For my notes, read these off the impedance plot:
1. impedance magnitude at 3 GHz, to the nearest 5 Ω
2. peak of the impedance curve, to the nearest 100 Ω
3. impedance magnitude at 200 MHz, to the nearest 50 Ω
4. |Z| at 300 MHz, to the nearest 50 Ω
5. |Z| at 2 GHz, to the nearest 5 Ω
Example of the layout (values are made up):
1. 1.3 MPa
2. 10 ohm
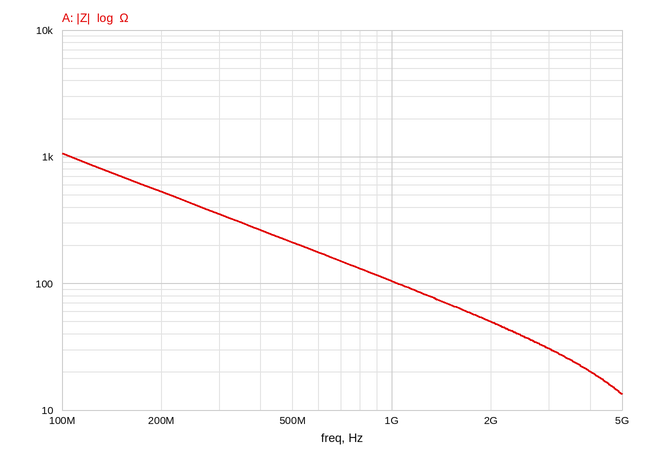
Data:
1. 30 Ω
2. 1.1 kΩ
3. 550 Ω
4. 350 Ω
5. 50 Ω
